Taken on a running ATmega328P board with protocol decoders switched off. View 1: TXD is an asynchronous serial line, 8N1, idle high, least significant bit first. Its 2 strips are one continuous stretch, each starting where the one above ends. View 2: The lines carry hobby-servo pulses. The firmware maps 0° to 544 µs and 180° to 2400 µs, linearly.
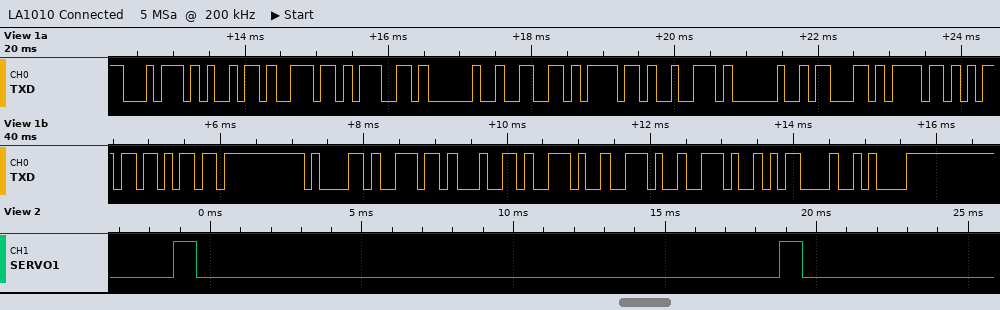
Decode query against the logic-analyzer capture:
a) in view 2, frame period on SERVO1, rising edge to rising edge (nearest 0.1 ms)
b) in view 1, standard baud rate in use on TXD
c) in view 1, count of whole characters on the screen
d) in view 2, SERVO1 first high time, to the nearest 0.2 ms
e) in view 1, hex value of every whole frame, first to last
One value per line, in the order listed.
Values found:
20.0 ms
9600 baud
21
0.8 ms
0x74 0x69 0x6E 0x67 0x20 0x66 0x6F 0x72 0x20 0x63 0x6F 0x6D 0x6D 0x61 0x6E 0x64 0x2E 0x2E 0x2E 0x0D 0x0A
